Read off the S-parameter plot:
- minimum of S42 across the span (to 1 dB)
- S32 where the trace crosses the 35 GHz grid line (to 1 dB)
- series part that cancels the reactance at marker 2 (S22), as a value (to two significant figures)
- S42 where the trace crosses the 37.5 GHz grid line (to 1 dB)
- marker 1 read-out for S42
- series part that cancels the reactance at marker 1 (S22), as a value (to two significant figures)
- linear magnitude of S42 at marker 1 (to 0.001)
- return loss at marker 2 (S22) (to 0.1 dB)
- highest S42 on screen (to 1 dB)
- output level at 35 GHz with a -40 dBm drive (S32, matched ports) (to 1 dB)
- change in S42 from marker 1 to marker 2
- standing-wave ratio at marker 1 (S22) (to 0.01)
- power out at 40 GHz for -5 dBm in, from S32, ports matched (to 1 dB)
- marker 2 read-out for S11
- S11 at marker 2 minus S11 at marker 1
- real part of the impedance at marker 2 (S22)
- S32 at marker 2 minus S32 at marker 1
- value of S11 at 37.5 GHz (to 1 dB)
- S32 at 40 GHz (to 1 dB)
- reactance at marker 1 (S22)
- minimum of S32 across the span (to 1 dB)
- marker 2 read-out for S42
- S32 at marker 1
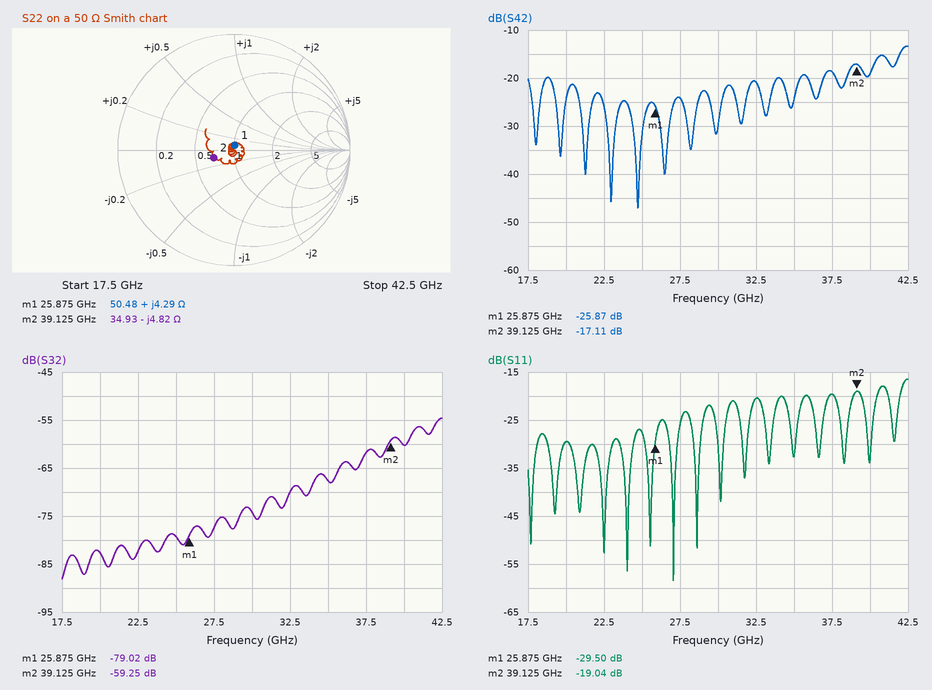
-47 dB
-68 dB
20 pH
-19 dB
-25.87 dB
1.4 pF
0.051
14.6 dB
-13 dB
-108 dBm
8.76 dB
1.09
-65 dBm
-19.04 dB
10.46 dB
34.93 Ω
19.77 dB
-20 dB
-60 dB
+4.29 Ω
-88 dB
-17.11 dB
-79.02 dB
